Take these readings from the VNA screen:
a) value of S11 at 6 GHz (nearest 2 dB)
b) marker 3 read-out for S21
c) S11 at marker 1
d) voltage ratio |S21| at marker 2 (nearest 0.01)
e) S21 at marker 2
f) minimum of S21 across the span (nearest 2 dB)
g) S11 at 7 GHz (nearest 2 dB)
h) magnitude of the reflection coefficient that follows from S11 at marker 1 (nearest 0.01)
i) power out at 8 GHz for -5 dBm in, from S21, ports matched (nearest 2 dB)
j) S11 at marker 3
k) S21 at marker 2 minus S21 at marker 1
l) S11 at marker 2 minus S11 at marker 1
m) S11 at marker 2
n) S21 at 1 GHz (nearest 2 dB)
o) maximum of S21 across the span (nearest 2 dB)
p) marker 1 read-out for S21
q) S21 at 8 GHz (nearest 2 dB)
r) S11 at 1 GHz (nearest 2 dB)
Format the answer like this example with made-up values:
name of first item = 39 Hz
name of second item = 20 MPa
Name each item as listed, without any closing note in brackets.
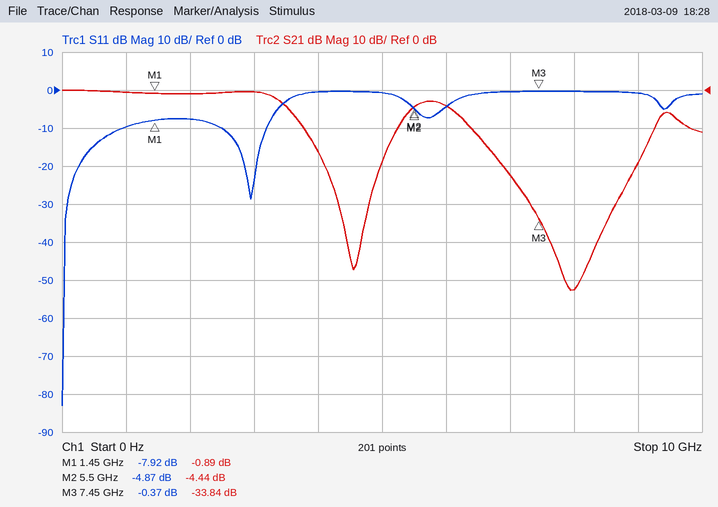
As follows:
value of S11 at 6 GHz = -4 dB
marker 3 read-out for S21 = -33.84 dB
S11 at marker 1 = -7.92 dB
voltage ratio |S21| at marker 2 = 0.60
S21 at marker 2 = -4.44 dB
minimum of S21 across the span = -52 dB
S11 at 7 GHz = 0 dB
magnitude of the reflection coefficient that follows from S11 at marker 1 = 0.40
power out at 8 GHz for -5 dBm in, from S21, ports matched = -58 dBm
S11 at marker 3 = -0.37 dB
S21 at marker 2 minus S21 at marker 1 = -3.55 dB
S11 at marker 2 minus S11 at marker 1 = 3.05 dB
S11 at marker 2 = -4.87 dB
S21 at 1 GHz = 0 dB
maximum of S21 across the span = 0 dB
marker 1 read-out for S21 = -0.89 dB
S21 at 8 GHz = -52 dB
S11 at 1 GHz = -10 dB
